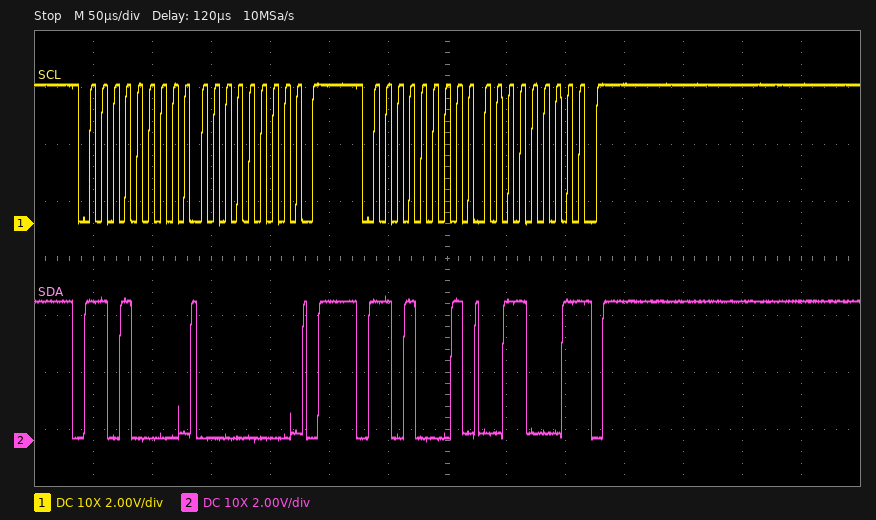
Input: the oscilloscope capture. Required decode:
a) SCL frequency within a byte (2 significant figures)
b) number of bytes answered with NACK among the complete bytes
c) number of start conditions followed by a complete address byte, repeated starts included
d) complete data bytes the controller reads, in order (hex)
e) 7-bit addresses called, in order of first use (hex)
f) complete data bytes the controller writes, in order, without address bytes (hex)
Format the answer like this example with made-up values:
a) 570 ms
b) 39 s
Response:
a) 100 kHz
b) 1
c) 2
d) 31
e) 0x68
f) 00
